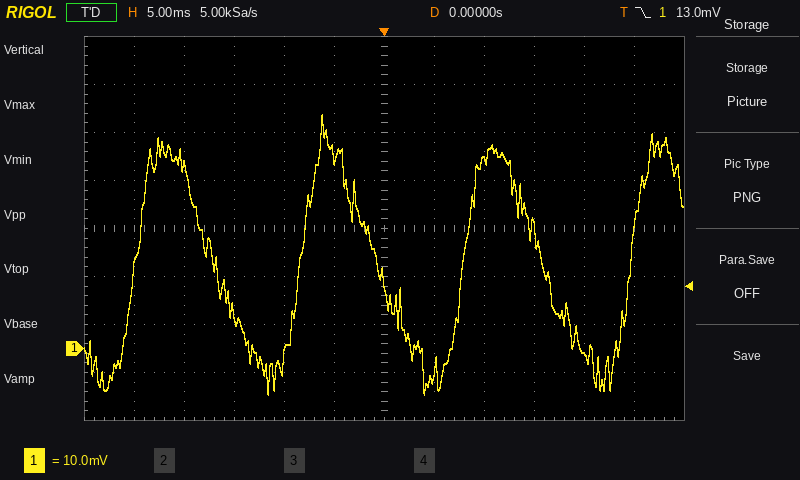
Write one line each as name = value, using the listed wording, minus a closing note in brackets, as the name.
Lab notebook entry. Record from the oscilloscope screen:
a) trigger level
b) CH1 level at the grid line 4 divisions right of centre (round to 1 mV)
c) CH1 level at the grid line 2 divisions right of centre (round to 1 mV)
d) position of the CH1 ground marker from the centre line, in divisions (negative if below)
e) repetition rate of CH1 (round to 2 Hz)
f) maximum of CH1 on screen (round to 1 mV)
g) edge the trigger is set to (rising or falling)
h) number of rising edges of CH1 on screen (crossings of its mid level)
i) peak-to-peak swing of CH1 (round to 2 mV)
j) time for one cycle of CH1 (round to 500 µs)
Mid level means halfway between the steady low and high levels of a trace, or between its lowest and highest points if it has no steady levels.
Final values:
trigger level = 13.0 mV
CH1 level at the grid line 4 divisions right of centre = -1 mV
CH1 level at the grid line 2 divisions right of centre = 39 mV
position of the CH1 ground marker from the centre line, in divisions = -2.5 div
repetition rate of CH1 = 60 Hz
maximum of CH1 on screen = 49 mV
edge the trigger is set to = falling
number of rising edges of CH1 on screen = 4
peak-to-peak swing of CH1 = 58 mV
time for one cycle of CH1 = 16.5 ms
